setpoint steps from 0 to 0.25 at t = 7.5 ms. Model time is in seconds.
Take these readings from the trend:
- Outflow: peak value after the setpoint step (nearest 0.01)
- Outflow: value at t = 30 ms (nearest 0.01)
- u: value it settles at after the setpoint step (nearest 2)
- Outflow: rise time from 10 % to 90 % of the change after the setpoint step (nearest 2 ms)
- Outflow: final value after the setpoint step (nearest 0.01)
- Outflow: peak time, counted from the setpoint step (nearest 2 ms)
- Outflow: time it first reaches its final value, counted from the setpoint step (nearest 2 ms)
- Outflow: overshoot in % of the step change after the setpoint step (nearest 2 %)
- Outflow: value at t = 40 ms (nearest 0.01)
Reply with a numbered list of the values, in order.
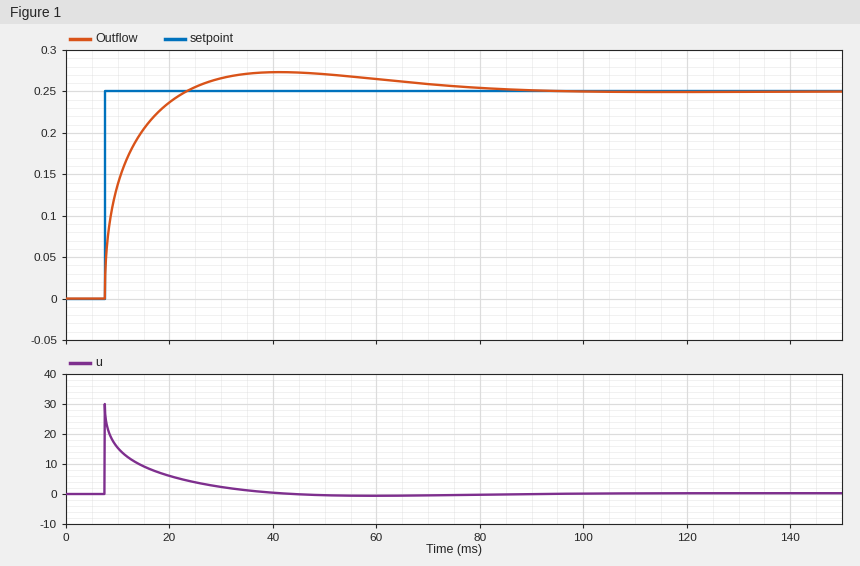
1. 0.27
2. 0.27
3. 0
4. 10 ms
5. 0.25
6. 34 ms
7. 16 ms
8. 10 %
9. 0.27
